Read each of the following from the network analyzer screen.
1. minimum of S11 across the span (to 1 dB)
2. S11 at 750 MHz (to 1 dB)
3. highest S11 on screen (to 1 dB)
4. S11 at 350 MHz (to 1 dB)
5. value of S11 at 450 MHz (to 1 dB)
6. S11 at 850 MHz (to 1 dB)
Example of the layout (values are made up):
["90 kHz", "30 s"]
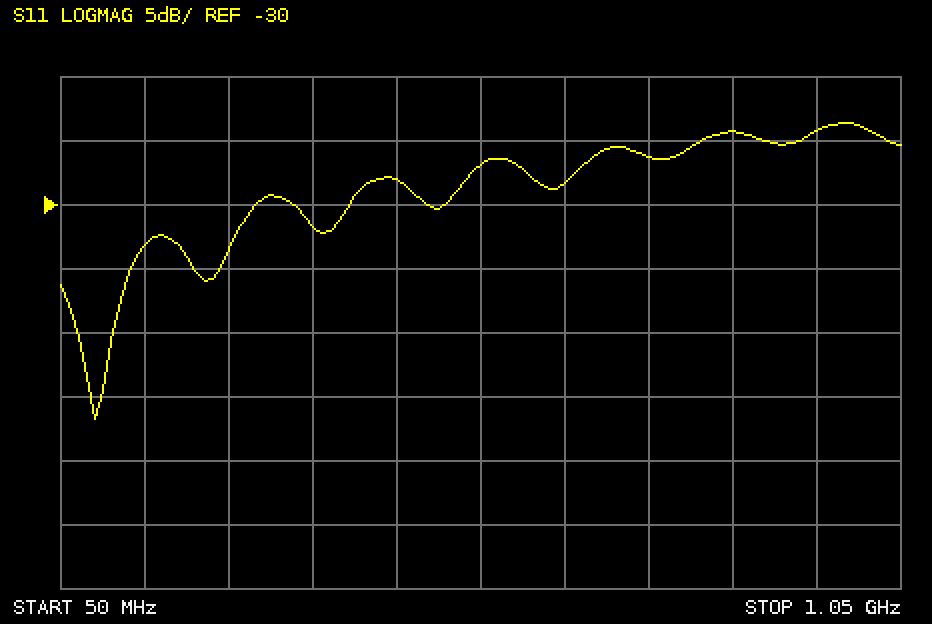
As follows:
["-47 dB", "-26 dB", "-24 dB", "-32 dB", "-28 dB", "-24 dB"]
